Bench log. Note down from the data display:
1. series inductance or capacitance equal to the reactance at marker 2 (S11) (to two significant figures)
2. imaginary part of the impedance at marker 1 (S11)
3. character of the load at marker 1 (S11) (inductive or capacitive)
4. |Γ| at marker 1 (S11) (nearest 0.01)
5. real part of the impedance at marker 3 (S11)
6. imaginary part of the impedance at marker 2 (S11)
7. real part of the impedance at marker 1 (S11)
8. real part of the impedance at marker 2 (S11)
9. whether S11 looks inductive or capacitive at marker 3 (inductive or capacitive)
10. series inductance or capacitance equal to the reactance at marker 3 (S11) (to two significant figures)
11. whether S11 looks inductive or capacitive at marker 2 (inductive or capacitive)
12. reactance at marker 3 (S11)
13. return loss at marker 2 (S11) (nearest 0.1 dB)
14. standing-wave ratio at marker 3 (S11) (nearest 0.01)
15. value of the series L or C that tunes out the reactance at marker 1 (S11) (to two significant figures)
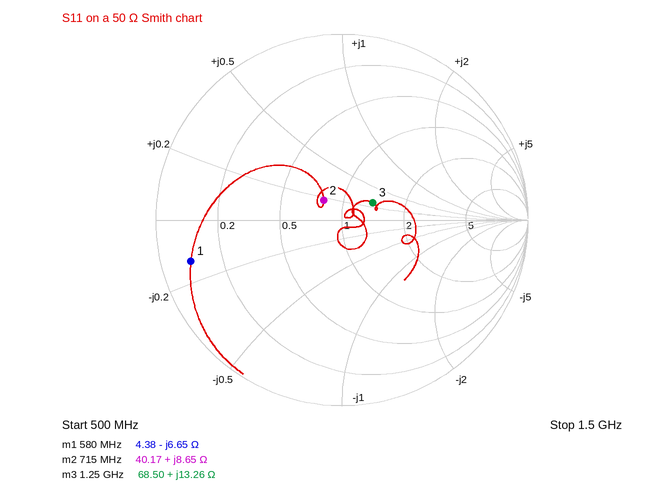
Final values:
1.9 nH
-6.65 Ω
capacitive
0.84
68.50 Ω
+8.65 Ω
4.38 Ω
40.17 Ω
inductive
1.7 nH
inductive
+13.26 Ω
16.8 dB
1.47
1.8 nH
